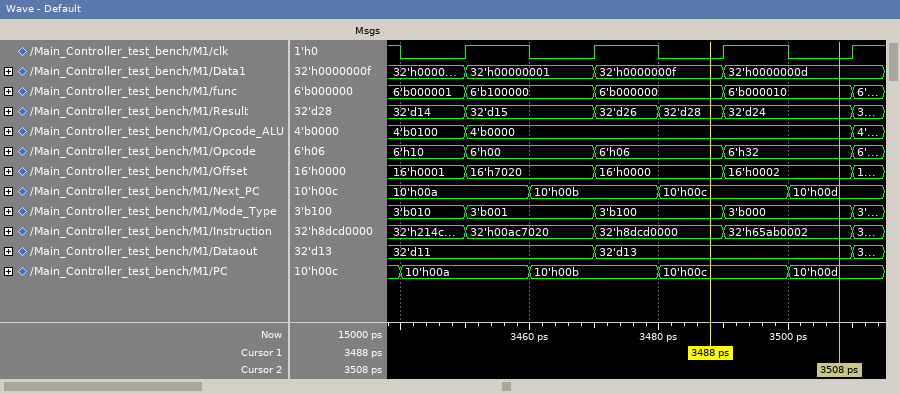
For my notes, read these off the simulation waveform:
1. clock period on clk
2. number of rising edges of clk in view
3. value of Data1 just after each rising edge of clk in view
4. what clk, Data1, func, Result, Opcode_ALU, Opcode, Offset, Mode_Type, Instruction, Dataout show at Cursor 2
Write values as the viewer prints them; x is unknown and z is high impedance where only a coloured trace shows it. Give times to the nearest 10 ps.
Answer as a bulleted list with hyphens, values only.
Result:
- 20 ps
- 4
- 32'h00000001, 32'h0000000f, 32'h0000000d, 32'h0000000d
- clk=0, Data1=32'h0000000d, func=6'b000010, Result=32'd24, Opcode_ALU=4'b0000, Opcode=6'h32, Offset=16'h0002, Mode_Type=3'b000, Instruction=32'h65ab0002, Dataout=32'd13
